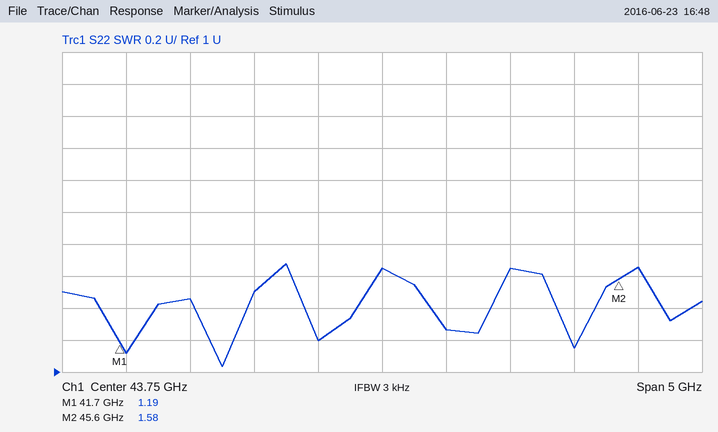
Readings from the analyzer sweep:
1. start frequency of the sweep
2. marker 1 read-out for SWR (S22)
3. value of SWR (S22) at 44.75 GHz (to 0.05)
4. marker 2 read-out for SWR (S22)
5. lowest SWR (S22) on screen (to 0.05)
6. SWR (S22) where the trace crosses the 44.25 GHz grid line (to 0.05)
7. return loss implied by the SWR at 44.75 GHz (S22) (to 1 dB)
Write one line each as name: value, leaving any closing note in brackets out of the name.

start frequency of the sweep: 41.25 GHz
marker 1 read-out for SWR: 1.19
value of SWR (S22) at 44.75 GHz: 1.65
marker 2 read-out for SWR: 1.58
lowest SWR (S22) on screen: 1.05
SWR (S22) where the trace crosses the 44.25 GHz grid line: 1.25
return loss implied by the SWR at 44.75 GHz (S22): 12 dB
